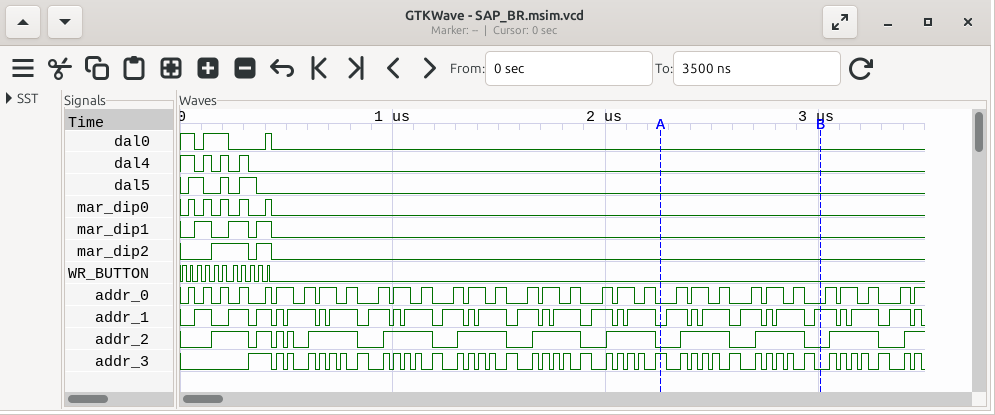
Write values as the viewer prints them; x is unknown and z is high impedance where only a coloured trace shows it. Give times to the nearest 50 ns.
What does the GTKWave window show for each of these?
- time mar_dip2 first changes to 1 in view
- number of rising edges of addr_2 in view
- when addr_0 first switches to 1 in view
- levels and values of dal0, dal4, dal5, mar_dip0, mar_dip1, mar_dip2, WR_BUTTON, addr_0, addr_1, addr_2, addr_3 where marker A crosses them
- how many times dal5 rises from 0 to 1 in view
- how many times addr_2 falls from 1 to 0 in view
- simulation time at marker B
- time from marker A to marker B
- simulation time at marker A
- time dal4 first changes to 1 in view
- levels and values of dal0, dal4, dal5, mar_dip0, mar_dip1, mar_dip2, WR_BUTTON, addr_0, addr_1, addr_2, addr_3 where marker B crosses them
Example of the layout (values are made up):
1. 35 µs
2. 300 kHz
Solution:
1. 150 ns
2. 13
3. 50 ns
4. dal0=0, dal4=0, dal5=0, mar_dip0=0, mar_dip1=0, mar_dip2=0, WR_BUTTON=0, addr_0=0, addr_1=0, addr_2=0, addr_3=1
5. 3
6. 12
7. 3000 ns
8. 750 ns
9. 2250 ns
10. 100 ns
11. dal0=0, dal4=0, dal5=0, mar_dip0=0, mar_dip1=0, mar_dip2=0, WR_BUTTON=0, addr_0=0, addr_1=1, addr_2=0, addr_3=0
